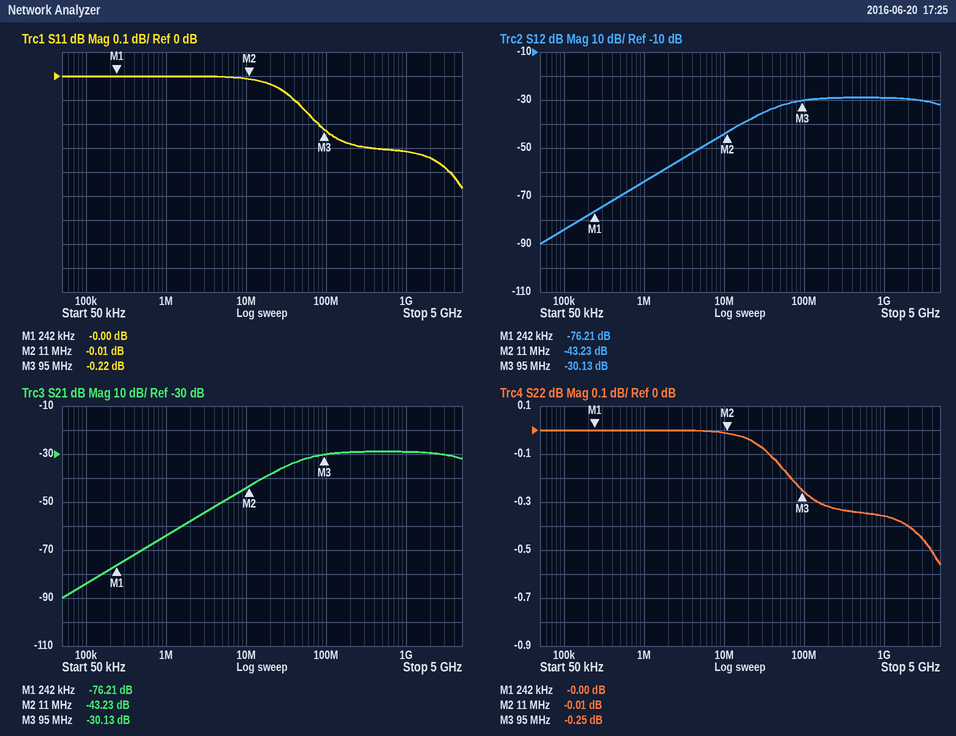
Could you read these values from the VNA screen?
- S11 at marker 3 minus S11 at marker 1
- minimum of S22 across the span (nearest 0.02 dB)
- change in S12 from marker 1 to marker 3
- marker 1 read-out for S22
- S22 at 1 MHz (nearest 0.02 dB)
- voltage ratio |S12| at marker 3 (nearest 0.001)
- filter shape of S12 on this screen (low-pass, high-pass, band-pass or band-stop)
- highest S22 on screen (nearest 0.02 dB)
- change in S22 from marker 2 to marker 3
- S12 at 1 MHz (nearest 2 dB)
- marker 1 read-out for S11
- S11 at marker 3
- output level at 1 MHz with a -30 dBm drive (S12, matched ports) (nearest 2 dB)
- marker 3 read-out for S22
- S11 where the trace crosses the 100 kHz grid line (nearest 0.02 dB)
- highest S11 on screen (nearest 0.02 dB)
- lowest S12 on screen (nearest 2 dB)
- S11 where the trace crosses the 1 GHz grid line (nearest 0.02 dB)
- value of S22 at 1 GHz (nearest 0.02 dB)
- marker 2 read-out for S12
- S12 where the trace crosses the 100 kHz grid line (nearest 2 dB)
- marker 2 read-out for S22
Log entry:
-0.22 dB
-0.56 dB
46.08 dB
-0.00 dB
0.00 dB
0.031
high-pass
0.00 dB
-0.24 dB
-64 dB
-0.00 dB
-0.22 dB
-94 dBm
-0.25 dB
0.00 dB
0.00 dB
-90 dB
-0.32 dB
-0.36 dB
-43.23 dB
-84 dB
-0.01 dB
